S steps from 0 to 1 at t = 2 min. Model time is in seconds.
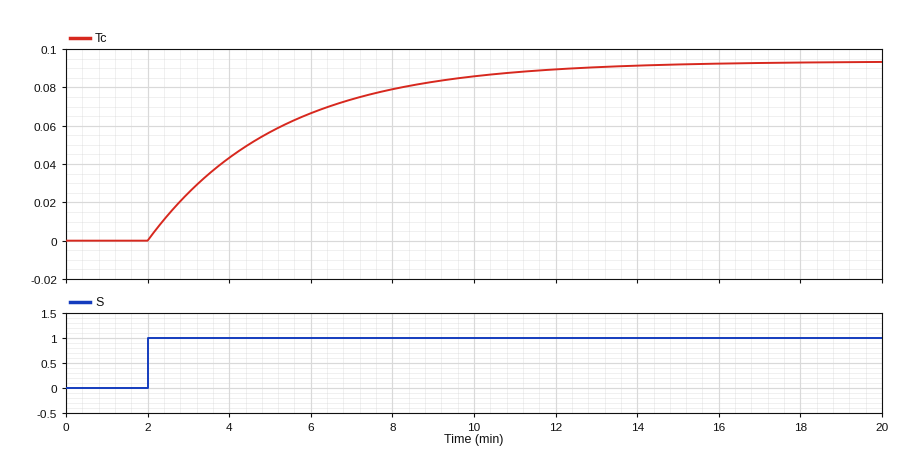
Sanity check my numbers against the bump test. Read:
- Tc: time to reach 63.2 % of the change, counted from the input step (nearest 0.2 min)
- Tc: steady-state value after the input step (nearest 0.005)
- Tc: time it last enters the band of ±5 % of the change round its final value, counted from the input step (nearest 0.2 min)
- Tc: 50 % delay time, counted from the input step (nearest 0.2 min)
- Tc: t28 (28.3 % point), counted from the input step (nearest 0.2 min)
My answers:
3.2 min
0.095
9.6 min
2.2 min
1.0 min
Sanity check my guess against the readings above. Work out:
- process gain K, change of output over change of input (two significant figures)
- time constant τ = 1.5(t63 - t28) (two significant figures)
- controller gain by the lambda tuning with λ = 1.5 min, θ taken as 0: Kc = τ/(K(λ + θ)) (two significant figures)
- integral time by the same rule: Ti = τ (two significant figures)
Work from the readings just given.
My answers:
0.095
3.3 min
23
3.3 min
